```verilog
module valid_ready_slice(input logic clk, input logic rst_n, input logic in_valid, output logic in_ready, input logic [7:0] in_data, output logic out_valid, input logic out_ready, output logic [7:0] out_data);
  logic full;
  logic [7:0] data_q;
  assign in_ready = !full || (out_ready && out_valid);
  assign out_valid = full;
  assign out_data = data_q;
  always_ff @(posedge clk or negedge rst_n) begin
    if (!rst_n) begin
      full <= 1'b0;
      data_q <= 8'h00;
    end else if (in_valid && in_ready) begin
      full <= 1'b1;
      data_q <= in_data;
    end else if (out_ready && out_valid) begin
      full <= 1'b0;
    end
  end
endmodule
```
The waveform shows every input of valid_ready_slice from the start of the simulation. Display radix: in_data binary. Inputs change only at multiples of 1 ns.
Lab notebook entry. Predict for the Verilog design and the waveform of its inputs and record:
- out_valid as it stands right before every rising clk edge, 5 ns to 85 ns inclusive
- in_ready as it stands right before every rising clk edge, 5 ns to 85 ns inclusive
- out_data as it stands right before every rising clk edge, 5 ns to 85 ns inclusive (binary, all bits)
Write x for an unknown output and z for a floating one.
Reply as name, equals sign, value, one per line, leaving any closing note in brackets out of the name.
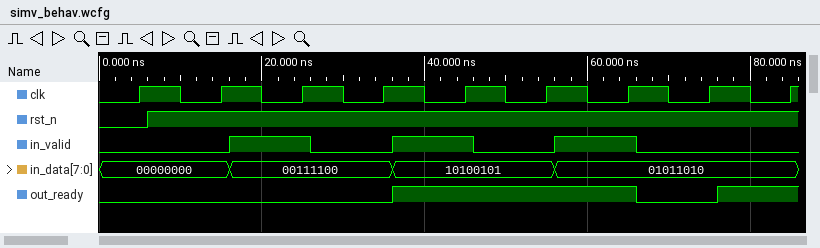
out_valid as it stands right before every rising clk edge, 5 ns to 85 ns inclusive = 0 0 0 1 1 1 0 1 1
in_ready as it stands right before every rising clk edge, 5 ns to 85 ns inclusive = 1 1 1 0 1 1 1 0 1
out_data as it stands right before every rising clk edge, 5 ns to 85 ns inclusive = 00000000, 00000000, 00000000, 00111100, 00111100, 10100101, 10100101, 01011010, 01011010
